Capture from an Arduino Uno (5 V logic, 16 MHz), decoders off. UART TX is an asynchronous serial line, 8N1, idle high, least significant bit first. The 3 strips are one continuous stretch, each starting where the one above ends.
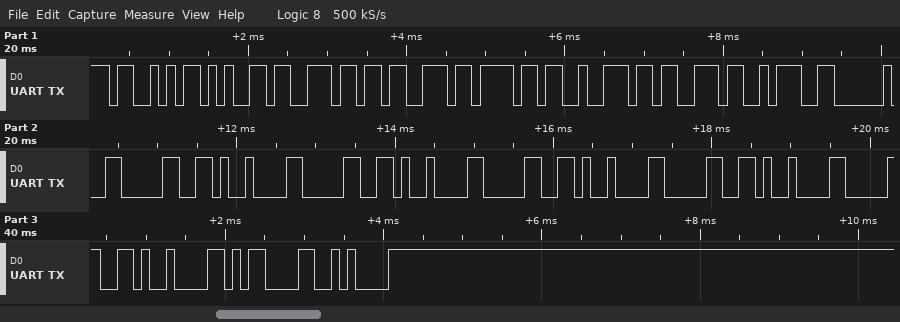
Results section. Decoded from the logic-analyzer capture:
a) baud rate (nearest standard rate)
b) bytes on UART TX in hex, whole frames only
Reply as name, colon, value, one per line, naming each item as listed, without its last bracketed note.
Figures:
baud rate: 9600 baud
bytes on UART TX in hex, whole frames only: 53 65 6E 73 6F 72 73 3A 20 30 09 30 09 30 09 30 09 30 09 0D 0A
